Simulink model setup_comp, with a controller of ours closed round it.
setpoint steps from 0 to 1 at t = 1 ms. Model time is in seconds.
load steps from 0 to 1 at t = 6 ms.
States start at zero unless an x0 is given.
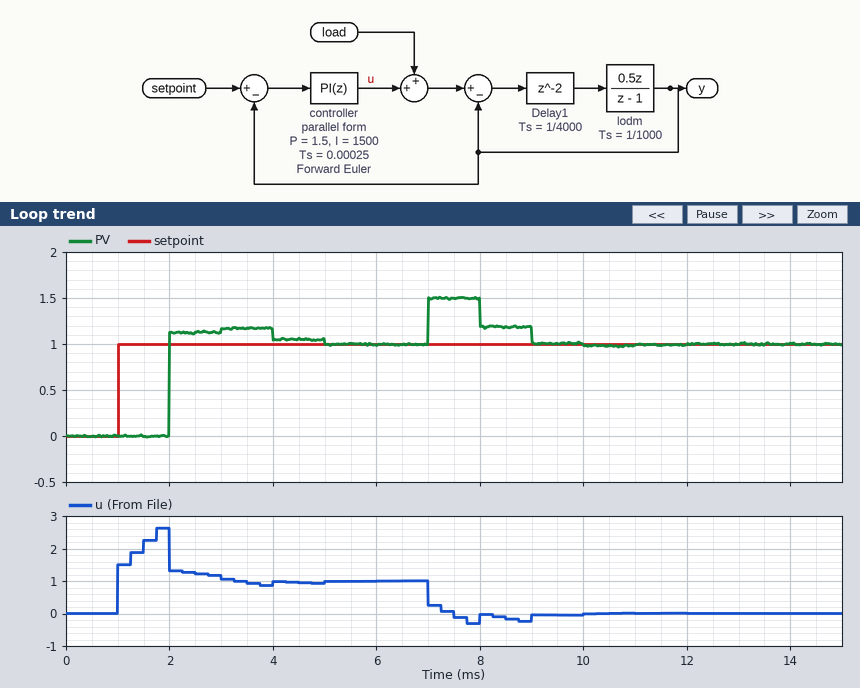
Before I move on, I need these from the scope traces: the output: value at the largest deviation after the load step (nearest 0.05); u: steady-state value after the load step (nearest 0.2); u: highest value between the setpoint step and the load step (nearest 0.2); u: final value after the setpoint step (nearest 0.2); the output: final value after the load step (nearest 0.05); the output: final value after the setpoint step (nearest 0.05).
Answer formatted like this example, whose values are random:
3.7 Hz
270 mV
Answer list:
1.50
0.0
2.6
1.0
1.00
1.00
